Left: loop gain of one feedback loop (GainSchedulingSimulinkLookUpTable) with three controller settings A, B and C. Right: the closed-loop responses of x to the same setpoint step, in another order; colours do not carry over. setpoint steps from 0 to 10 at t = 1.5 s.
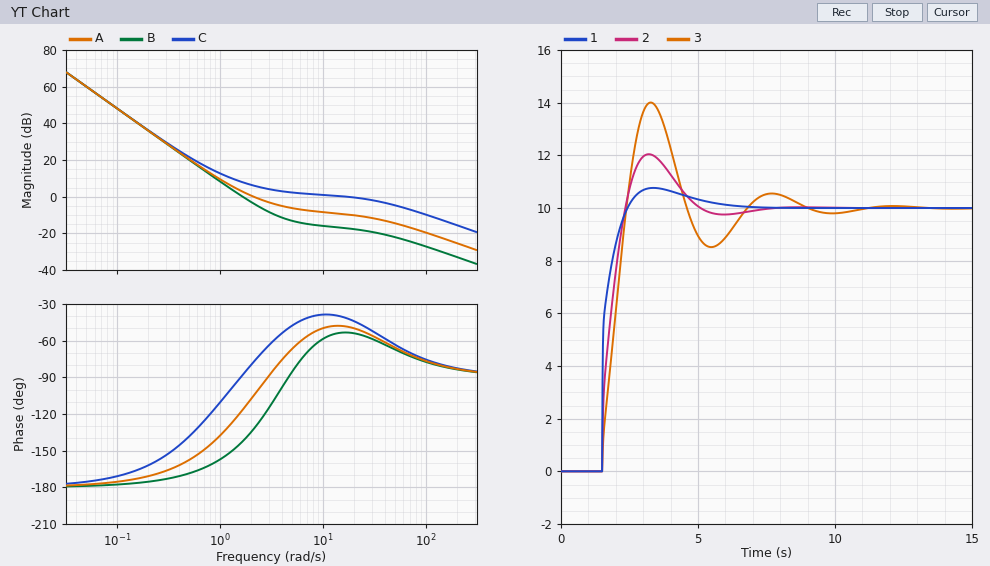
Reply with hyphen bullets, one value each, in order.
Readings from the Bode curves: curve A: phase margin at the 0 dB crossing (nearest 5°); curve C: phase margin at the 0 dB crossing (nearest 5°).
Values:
- 75°
- 140°
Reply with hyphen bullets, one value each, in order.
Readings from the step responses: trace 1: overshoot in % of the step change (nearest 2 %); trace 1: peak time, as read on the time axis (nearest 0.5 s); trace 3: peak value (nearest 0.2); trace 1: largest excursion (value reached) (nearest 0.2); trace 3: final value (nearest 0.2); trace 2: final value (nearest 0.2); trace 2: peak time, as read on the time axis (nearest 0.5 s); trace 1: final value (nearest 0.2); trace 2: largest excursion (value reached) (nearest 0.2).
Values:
- 8 %
- 3.5 s
- 14.0
- 10.8
- 10.0
- 10.0
- 3.0 s
- 10.0
- 12.0
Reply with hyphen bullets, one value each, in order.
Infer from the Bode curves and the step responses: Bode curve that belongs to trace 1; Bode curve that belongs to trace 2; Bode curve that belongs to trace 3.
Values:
- C
- A
- B
